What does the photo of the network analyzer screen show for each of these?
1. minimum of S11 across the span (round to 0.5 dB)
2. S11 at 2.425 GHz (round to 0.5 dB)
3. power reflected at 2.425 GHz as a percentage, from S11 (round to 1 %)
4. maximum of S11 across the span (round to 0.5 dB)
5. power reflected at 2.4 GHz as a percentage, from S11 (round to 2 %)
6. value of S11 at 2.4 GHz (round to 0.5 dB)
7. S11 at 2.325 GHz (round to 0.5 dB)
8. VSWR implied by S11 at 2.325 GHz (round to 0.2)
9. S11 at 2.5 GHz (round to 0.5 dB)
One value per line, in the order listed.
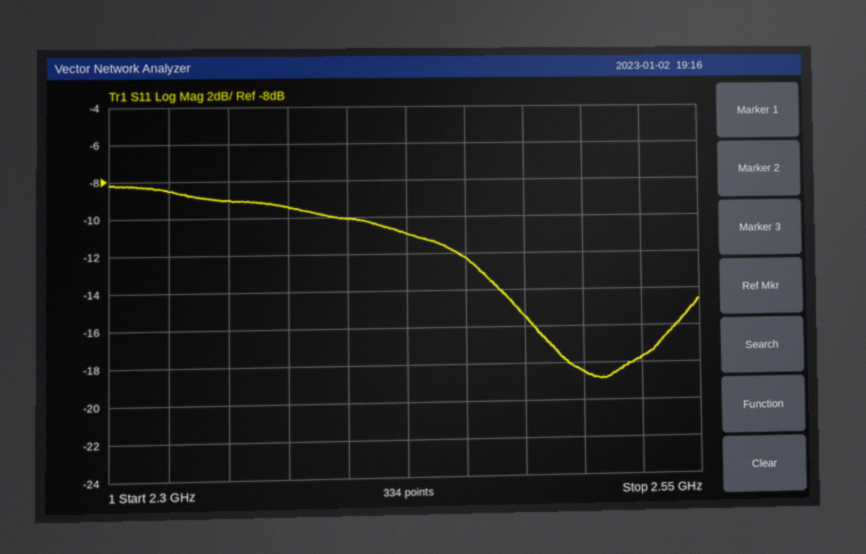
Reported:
-19.0 dB
-11.0 dB
8 %
-8.0 dB
10 %
-10.0 dB
-8.5 dB
2.2
-18.5 dB
